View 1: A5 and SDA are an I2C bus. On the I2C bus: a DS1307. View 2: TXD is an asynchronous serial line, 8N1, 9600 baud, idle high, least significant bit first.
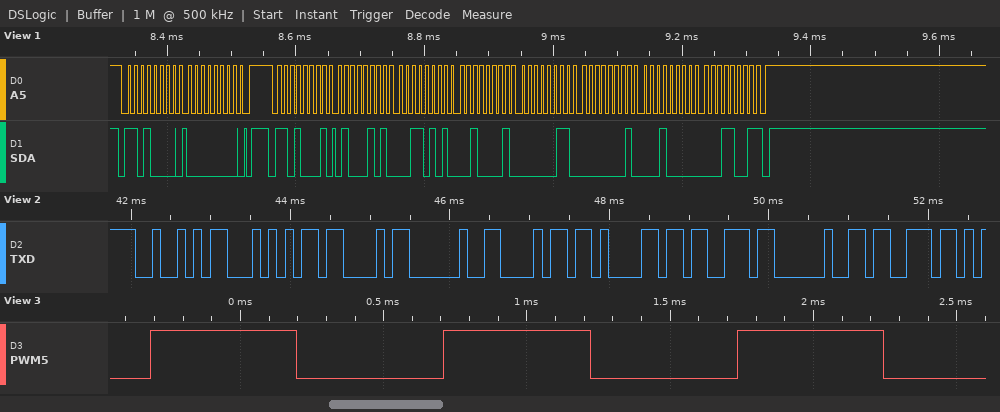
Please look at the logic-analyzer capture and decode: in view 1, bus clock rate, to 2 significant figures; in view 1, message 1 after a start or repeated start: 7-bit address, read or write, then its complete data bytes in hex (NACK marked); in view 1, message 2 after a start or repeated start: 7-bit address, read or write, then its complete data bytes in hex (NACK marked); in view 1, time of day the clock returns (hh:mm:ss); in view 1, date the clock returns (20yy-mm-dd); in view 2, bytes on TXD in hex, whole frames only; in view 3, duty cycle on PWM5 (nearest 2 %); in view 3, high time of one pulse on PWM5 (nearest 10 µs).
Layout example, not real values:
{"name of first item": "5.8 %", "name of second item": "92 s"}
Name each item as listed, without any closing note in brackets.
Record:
{"in view 1, bus clock rate, to 2 significant figures": "100 kHz", "in view 1, message 1 after a start or repeated start: 7-bit address, read or write, then its complete data bytes in hex": "0x68 write: 00", "in view 1, message 2 after a start or repeated start: 7-bit address, read or write, then its complete data bytes in hex": "0x68 read: 45 35 21 03 01 10 19 NACK", "in view 1, time of day the clock returns": "21:35:45", "in view 1, date the clock returns": "2019-10-01", "in view 2, bytes on TXD in hex, whole frames only": "52 54 43 20 68 61 73 20 73", "in view 3, duty cycle on PWM5": "50 %", "in view 3, high time of one pulse on PWM5": "510 µs"}
